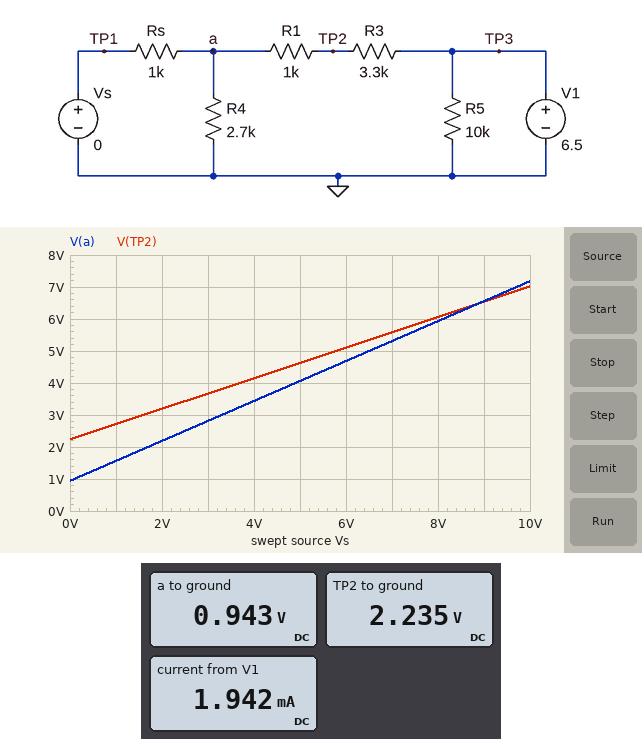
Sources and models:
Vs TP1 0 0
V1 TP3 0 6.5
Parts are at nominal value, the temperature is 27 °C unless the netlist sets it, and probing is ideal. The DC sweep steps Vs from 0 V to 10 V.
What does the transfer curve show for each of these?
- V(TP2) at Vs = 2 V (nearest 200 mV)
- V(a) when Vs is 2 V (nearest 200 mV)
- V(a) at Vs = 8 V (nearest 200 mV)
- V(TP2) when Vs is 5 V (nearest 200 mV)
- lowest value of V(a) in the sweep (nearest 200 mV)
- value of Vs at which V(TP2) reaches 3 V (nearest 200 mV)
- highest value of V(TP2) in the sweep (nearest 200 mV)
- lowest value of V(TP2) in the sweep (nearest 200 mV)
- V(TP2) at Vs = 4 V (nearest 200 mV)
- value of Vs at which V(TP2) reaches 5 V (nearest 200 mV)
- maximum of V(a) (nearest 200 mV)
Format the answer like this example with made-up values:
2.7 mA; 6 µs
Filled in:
3.2 V; 2.2 V; 6.0 V; 4.6 V; 1.0 V; 1.6 V; 7.0 V; 2.2 V; 4.2 V; 5.8 V; 7.2 V
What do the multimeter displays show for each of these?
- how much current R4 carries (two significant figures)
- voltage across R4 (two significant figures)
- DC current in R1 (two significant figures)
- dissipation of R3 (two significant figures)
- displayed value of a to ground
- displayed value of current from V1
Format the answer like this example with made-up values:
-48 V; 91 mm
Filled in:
350 µA; 940 mV; 1.3 mA; 5.5 mW; 0.943 V; 1.942 mA
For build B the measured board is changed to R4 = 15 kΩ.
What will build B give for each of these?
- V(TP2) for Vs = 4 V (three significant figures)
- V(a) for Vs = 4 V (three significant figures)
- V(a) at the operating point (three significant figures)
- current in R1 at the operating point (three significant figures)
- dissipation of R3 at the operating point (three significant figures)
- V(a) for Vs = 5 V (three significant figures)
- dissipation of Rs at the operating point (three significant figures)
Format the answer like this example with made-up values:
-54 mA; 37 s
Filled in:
4.77 V; 4.24 V; 1.16 V; 1.24 mA; 5.08 mW; 5.01 V; 1.35 mW
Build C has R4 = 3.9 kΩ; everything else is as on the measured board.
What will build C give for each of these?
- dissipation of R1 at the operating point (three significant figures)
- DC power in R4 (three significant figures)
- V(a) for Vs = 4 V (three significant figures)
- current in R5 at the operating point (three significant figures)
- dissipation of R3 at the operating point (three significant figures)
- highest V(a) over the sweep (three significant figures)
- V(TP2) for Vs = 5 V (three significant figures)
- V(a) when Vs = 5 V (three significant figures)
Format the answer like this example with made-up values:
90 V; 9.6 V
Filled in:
1.63 mW; 264 µW; 3.70 V; 650 µA; 5.37 mW; 7.73 V; 4.87 V; 4.37 V
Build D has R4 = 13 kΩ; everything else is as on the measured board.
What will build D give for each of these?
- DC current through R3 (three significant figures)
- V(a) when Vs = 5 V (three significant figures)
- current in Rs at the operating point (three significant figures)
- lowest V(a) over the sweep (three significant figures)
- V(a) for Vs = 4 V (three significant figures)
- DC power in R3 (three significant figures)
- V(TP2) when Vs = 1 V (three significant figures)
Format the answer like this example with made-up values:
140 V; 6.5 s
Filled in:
1.24 mA; 4.97 V; 1.15 mA; 1.15 V; 4.21 V; 5.10 mW; 2.98 V
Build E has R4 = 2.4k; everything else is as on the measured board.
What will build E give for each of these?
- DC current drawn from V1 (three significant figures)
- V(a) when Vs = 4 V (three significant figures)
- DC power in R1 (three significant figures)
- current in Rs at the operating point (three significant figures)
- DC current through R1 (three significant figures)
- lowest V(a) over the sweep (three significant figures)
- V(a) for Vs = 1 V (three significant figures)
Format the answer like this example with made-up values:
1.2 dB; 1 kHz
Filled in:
1.95 mA; 3.34 V; 1.69 mW; 917 µA; 1.30 mA; 917 mV; 1.52 V
